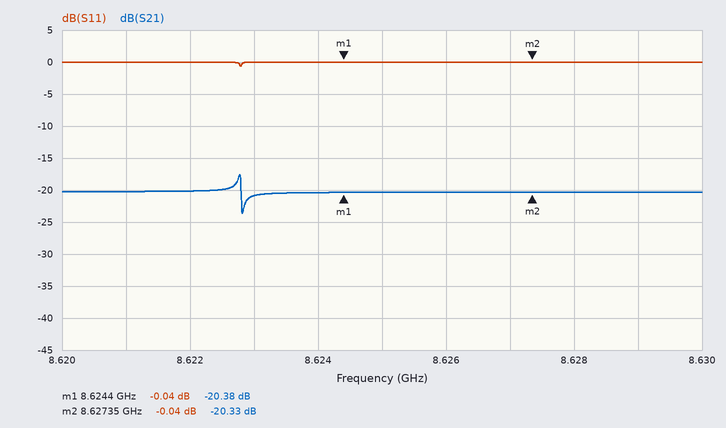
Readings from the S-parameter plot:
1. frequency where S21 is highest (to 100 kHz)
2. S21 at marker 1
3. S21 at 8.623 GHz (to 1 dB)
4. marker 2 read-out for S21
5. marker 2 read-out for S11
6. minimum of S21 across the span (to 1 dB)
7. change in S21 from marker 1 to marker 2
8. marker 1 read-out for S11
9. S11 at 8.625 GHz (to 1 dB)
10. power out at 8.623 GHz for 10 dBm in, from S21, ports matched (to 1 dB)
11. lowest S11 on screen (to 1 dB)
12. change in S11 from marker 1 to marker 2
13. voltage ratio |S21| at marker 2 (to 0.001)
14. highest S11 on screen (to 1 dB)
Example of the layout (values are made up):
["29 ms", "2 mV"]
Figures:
["8.6228 GHz", "-20.38 dB", "-21 dB", "-20.33 dB", "-0.04 dB", "-24 dB", "0.05 dB", "-0.04 dB", "0 dB", "-11 dBm", "-1 dB", "0.00 dB", "0.096", "0 dB"]
